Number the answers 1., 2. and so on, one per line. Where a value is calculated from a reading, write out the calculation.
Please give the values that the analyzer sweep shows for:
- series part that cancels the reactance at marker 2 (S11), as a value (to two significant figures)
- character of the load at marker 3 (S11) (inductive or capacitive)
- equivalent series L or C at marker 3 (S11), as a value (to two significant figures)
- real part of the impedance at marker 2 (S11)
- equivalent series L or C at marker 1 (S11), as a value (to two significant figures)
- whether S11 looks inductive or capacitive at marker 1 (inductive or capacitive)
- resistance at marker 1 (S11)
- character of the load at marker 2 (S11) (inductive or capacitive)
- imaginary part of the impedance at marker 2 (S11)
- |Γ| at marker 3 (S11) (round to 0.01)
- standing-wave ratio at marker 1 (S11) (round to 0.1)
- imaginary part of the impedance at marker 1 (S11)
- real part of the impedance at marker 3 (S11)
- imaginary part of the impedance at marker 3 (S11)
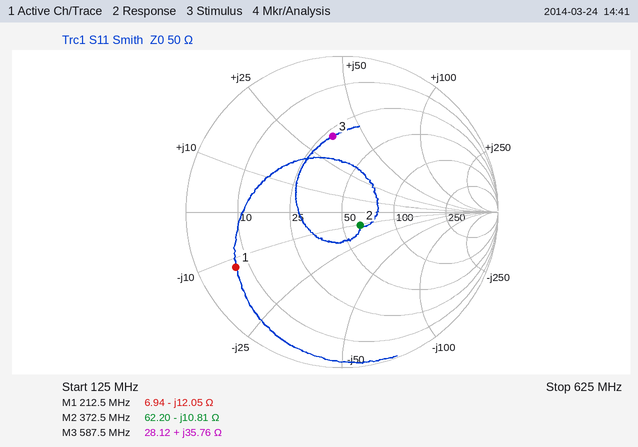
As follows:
1. L = 10.81 Ω/(2π × 372.5 MHz) ≈ 4.6 nH
2. inductive
3. L = 35.76 Ω/(2π × 587.5 MHz) ≈ 9.7 nH
4. 62.20 Ω
5. C = 1/(2π × 212.5 MHz × 12.05 Ω) ≈ 62 pF
6. capacitive
7. 6.94 Ω
8. capacitive
9. -10.81 Ω
10. 0.49
11. 7.6
12. -12.05 Ω
13. 28.12 Ω
14. +35.76 Ω
